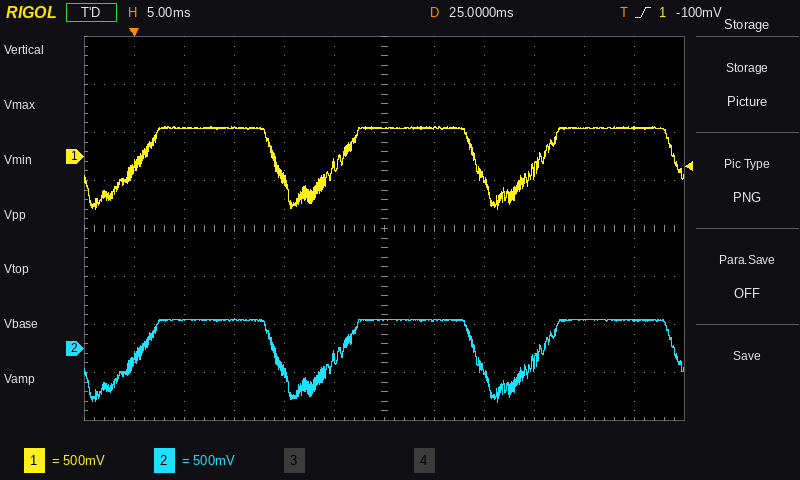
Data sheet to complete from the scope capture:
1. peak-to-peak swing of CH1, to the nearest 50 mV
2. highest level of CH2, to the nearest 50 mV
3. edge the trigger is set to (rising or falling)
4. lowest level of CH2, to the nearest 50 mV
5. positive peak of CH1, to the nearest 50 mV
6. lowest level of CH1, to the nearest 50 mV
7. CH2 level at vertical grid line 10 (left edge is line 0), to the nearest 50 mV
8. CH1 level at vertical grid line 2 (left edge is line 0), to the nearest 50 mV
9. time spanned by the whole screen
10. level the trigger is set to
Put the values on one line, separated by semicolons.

850 mV; 300 mV; rising; -550 mV; 300 mV; -550 mV; 300 mV; 300 mV; 60 ms; -100 mV
